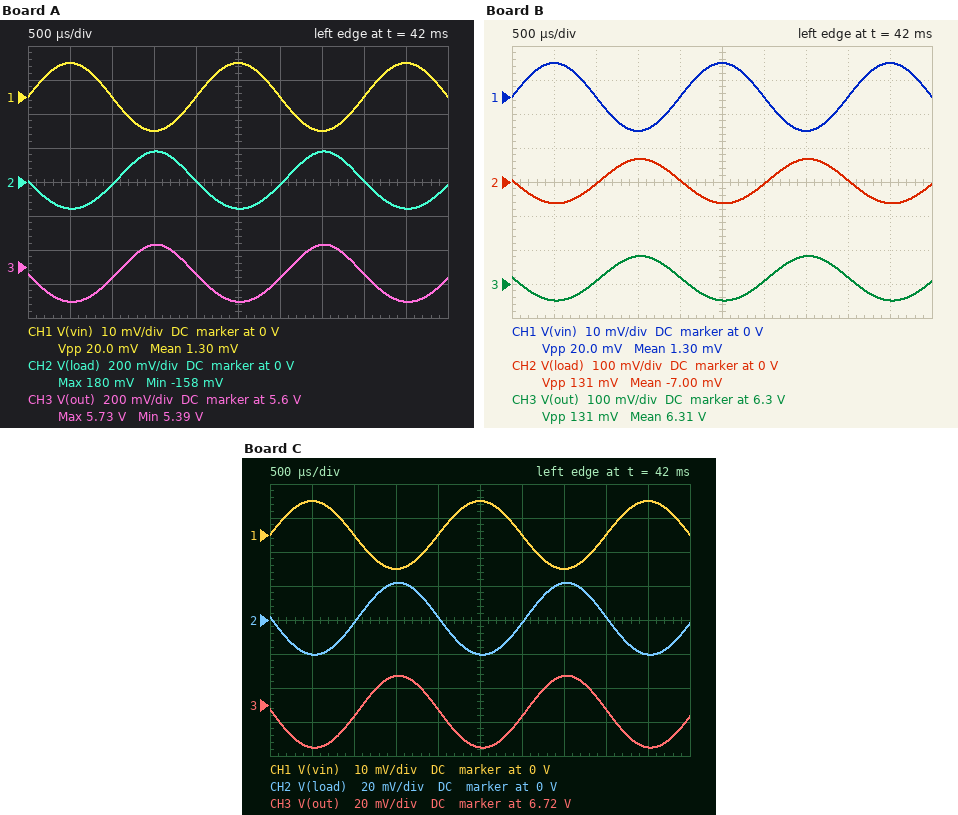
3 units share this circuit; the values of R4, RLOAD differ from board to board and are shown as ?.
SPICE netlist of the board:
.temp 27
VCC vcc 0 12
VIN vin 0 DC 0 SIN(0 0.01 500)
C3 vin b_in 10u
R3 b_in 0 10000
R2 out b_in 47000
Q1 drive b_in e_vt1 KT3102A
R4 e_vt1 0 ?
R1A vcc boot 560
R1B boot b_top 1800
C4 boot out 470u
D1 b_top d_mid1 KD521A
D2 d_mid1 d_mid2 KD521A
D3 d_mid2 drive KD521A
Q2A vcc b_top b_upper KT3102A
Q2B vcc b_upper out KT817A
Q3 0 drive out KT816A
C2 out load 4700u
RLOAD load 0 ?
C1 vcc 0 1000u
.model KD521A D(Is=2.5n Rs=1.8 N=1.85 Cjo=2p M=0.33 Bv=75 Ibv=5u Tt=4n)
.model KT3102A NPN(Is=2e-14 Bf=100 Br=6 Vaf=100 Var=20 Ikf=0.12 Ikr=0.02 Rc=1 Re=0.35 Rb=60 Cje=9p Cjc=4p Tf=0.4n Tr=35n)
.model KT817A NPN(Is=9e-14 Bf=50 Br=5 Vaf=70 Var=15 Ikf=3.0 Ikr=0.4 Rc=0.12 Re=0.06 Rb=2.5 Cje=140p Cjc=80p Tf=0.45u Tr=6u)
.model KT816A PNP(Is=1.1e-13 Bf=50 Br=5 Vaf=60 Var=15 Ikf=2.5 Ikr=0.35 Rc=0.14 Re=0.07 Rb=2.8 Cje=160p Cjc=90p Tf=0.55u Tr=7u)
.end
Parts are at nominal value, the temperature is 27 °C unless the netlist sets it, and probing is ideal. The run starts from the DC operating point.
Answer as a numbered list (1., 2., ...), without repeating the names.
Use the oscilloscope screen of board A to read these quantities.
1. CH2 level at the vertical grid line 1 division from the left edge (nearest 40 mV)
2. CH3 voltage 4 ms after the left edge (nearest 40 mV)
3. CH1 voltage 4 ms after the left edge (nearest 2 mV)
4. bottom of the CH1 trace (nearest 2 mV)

1. -160 mV
2. 5.56 V
3. 0 V
4. -10 mV
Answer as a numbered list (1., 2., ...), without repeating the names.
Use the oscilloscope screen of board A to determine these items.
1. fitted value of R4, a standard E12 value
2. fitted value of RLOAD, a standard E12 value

1. 33 Ω
2. 10 Ω
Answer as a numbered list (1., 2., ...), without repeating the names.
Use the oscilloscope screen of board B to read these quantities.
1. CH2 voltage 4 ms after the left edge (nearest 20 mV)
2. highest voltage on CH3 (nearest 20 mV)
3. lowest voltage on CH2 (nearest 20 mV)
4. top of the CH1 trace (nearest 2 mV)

1. 0 V
2. 6.38 V
3. -60 mV
4. 10 mV
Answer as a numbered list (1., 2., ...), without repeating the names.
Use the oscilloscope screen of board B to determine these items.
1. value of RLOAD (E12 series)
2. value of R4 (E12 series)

1. 12 Ω
2. 120 Ω
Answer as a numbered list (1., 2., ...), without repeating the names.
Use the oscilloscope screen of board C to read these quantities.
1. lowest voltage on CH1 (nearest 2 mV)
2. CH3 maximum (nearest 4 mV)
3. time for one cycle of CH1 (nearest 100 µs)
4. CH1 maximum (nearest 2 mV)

1. -10 mV
2. 6.736 V
3. 2.0 ms
4. 10 mV
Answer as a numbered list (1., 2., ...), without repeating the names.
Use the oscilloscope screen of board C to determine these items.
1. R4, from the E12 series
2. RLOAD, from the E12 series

1. 180 Ω
2. 5.6 Ω
